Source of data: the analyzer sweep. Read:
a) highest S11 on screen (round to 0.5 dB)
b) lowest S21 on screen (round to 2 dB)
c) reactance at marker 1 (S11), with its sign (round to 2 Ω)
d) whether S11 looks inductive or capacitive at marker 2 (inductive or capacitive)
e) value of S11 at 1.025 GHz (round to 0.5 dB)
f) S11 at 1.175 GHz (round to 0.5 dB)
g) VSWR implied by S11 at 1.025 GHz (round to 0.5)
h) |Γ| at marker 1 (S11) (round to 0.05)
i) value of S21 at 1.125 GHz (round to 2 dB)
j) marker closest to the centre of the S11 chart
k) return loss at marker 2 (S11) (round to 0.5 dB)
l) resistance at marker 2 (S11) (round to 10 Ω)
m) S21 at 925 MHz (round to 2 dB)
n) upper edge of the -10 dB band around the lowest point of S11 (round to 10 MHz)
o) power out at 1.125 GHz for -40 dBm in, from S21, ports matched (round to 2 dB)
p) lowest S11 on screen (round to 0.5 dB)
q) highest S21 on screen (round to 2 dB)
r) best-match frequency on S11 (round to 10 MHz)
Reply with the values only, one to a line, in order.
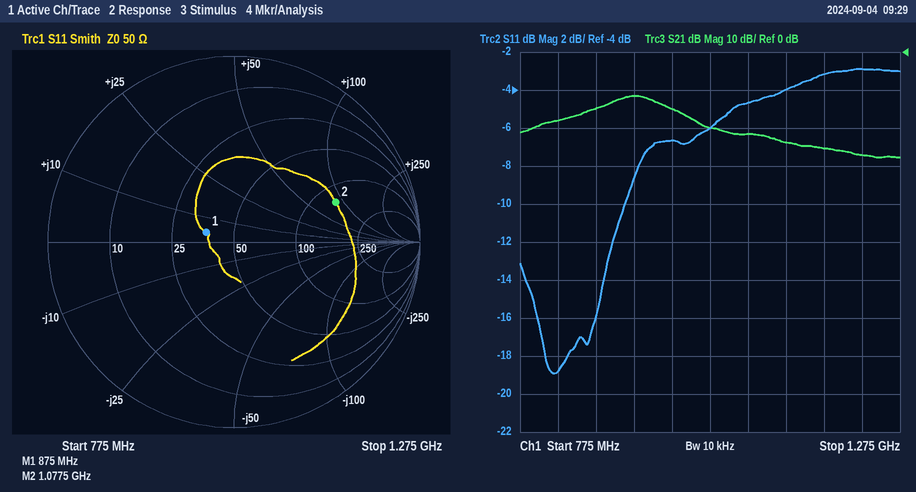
-3.0 dB
-28 dB
+4 Ω
inductive
-6.0 dB
-3.0 dB
3.0
0.15
-24 dB
marker 1
4.5 dB
130 Ω
-12 dB
910 MHz
-64 dBm
-19.0 dB
-12 dB
820 MHz
